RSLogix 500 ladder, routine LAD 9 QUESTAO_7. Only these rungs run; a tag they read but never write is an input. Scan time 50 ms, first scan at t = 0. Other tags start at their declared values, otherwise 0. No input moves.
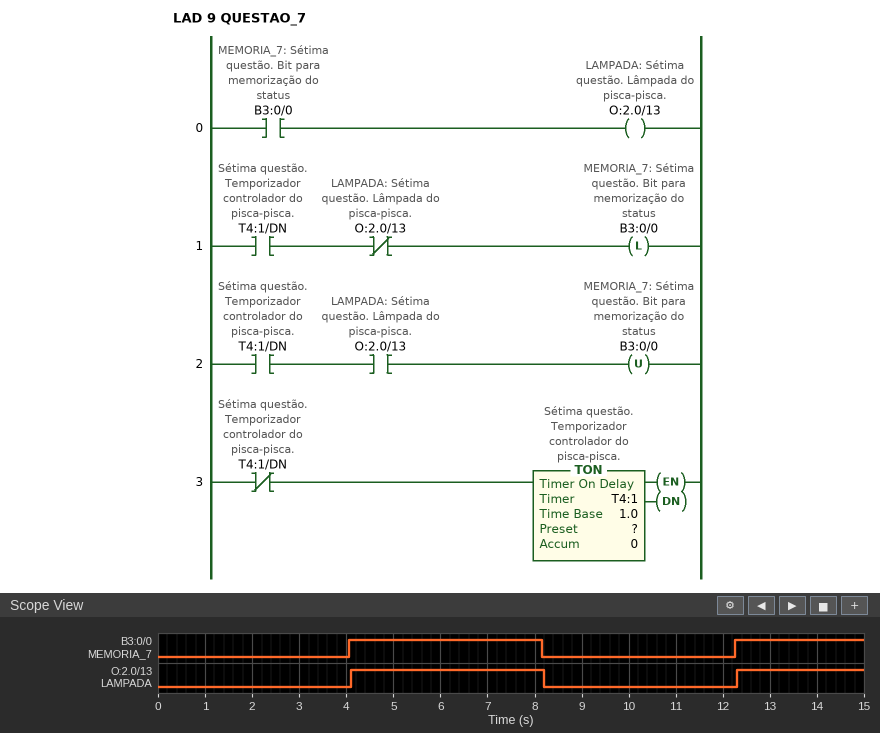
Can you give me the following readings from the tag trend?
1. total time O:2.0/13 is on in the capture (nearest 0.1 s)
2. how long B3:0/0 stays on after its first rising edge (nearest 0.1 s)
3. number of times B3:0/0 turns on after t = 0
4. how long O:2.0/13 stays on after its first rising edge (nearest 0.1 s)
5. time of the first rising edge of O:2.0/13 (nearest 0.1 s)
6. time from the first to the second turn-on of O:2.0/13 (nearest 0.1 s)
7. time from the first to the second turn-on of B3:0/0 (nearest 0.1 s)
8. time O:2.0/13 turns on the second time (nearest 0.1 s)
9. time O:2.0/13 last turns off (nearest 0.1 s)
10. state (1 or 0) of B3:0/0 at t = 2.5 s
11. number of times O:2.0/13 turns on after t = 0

6.8 s
4.1 s
2
4.1 s
4.1 s
8.2 s
8.2 s
12.3 s
8.2 s
0
2
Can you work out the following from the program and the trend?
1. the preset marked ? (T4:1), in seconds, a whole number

4 s
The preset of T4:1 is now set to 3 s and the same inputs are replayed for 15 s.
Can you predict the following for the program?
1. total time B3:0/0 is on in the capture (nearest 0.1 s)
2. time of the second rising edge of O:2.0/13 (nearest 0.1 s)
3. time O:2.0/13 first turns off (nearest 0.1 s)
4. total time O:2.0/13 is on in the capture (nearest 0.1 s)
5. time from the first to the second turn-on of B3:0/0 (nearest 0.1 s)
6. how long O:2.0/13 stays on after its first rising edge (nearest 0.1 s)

6.2 s
9.3 s
6.2 s
6.2 s
6.2 s
3.1 s
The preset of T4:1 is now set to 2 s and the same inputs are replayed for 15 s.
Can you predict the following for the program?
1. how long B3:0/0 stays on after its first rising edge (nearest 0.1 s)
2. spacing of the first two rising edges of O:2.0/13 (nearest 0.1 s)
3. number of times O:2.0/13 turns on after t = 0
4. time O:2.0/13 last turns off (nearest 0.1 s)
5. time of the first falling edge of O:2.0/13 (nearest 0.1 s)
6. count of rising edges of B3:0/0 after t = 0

2.1 s
4.2 s
4
12.6 s
4.2 s
4
